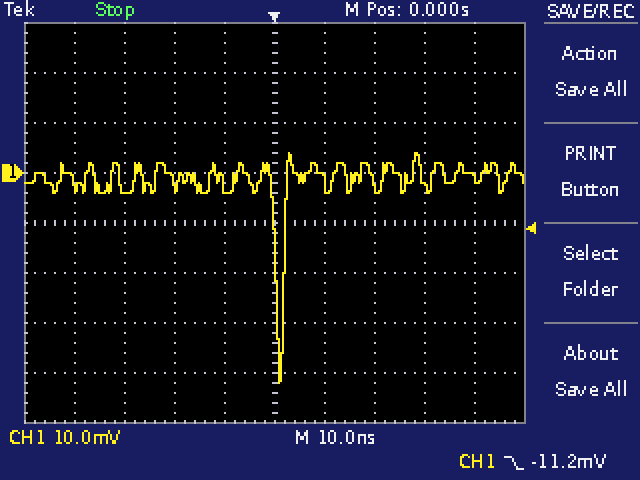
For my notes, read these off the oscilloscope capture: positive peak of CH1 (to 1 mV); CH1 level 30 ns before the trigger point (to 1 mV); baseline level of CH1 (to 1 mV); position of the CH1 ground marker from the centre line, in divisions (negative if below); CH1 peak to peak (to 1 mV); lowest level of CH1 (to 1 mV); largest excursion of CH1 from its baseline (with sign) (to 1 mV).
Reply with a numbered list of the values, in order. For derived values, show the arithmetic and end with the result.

1. 4 mV
2. -3 mV
3. -1 mV
4. +1.0 div
5. 4 mV − (-42 mV) = 46 mV
6. -42 mV
7. -42 mV − (-1 mV) = -41 mV
